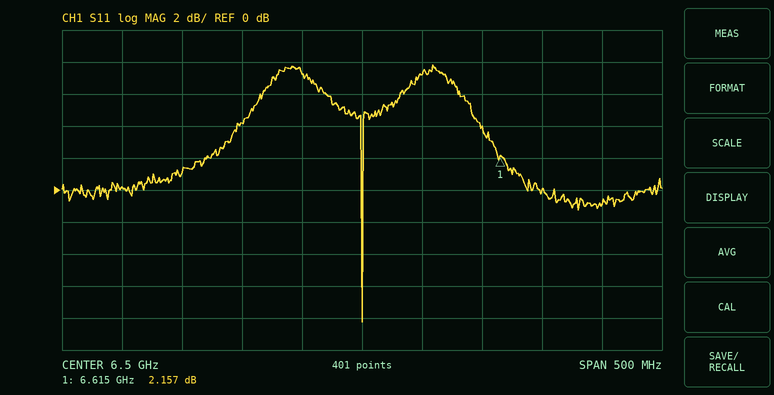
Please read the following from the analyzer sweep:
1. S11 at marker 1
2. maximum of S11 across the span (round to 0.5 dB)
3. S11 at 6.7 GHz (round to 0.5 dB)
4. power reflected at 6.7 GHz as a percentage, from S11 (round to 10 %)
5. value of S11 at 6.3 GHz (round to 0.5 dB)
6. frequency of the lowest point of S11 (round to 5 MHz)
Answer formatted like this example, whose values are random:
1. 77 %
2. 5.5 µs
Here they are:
1. 2.157 dB
2. 8.0 dB
3. -1.0 dB
4. 80 %
5. 0.0 dB
6. 6.500 GHz
